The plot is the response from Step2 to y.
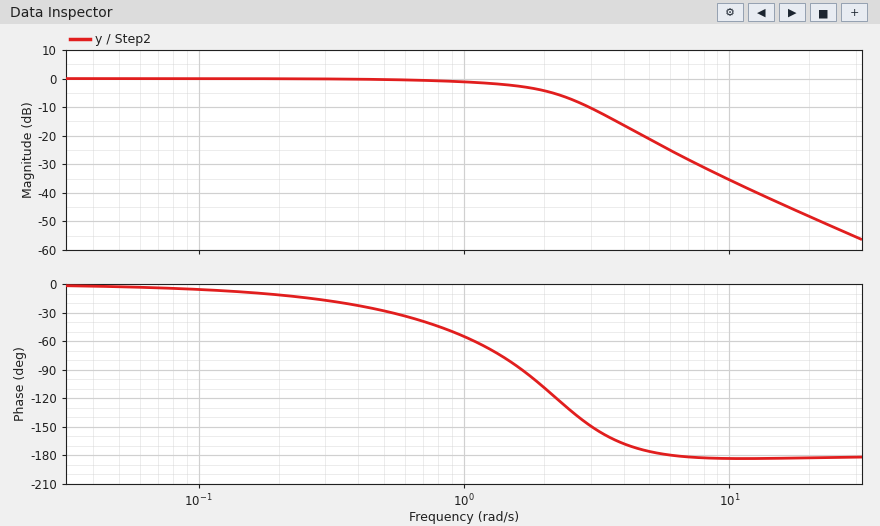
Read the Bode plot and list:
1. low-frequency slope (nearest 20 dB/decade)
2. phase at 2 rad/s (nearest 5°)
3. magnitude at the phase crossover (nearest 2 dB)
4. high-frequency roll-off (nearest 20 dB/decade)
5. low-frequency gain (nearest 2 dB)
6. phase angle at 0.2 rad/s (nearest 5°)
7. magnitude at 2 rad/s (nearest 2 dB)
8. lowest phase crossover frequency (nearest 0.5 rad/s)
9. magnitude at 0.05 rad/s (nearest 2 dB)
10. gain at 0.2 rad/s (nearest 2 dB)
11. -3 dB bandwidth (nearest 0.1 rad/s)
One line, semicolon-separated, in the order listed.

0 dB/decade; -110°; -26 dB; -40 dB/decade; 0 dB; -10°; -4 dB; 6.0 rad/s; 0 dB; 0 dB; 1.7 rad/s
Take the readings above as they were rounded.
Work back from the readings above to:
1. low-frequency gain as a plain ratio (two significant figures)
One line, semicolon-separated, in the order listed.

1.0
